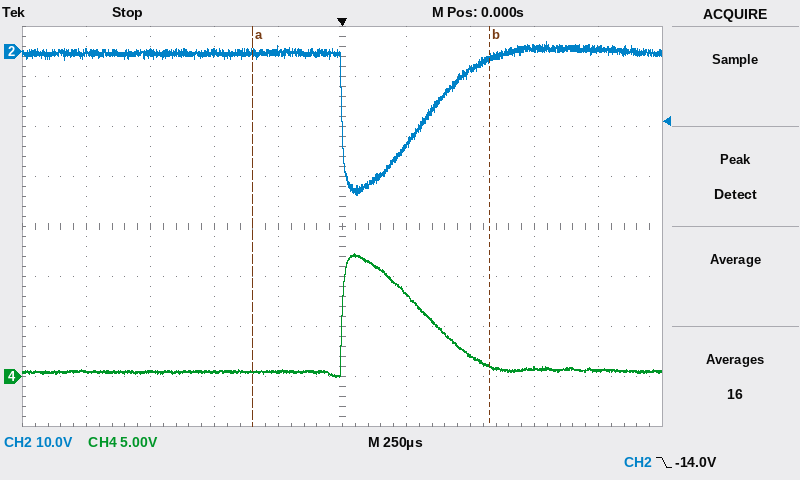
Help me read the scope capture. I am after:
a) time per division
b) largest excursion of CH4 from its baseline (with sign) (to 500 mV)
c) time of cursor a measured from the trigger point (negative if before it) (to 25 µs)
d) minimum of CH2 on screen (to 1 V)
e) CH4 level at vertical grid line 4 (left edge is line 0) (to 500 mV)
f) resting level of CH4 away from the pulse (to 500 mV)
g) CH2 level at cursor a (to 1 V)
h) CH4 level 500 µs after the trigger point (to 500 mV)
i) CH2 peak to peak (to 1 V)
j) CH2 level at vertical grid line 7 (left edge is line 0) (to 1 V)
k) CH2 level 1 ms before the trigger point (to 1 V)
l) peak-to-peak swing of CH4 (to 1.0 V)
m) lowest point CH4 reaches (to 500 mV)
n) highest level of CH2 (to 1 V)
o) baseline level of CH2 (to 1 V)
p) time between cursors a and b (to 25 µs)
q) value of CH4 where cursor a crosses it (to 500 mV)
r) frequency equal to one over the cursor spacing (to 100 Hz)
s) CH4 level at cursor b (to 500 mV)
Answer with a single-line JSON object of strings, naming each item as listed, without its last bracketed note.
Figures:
{"time per division": "250 µs", "largest excursion of CH4 from its baseline (with sign)": "+12.0 V", "time of cursor a measured from the trigger point (negative if before it)": "-350 µs", "minimum of CH2 on screen": "-29 V", "CH4 level at vertical grid line 4 (left edge is line 0)": "500 mV", "resting level of CH4 away from the pulse": "500 mV", "CH2 level at cursor a": "0 V", "CH4 level 500 µs after the trigger point": "2.0 V", "CH2 peak to peak": "31 V", "CH2 level at vertical grid line 7 (left edge is line 0)": "-4 V", "CH2 level 1 ms before the trigger point": "0 V", "peak-to-peak swing of CH4": "12.0 V", "lowest point CH4 reaches": "0.0 V", "highest level of CH2": "2 V", "baseline level of CH2": "0 V", "time between cursors a and b": "925 µs", "value of CH4 where cursor a crosses it": "500 mV", "frequency equal to one over the cursor spacing": "1.1 kHz", "CH4 level at cursor b": "1.0 V"}
